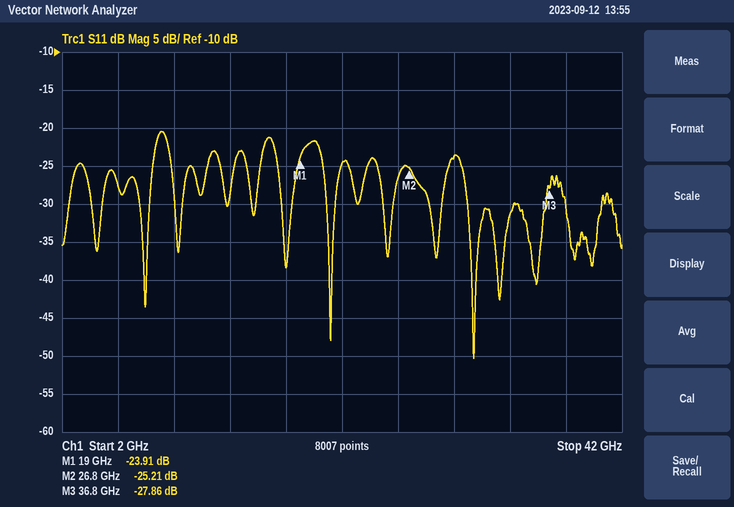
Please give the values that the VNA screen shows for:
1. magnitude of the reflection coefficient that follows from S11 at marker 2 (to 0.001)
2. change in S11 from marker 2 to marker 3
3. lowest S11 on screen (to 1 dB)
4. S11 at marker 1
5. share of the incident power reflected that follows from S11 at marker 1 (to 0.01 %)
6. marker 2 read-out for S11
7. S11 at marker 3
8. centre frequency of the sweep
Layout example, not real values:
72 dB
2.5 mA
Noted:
0.055
-2.65 dB
-50 dB
-23.91 dB
0.41 %
-25.21 dB
-27.86 dB
22 GHz
